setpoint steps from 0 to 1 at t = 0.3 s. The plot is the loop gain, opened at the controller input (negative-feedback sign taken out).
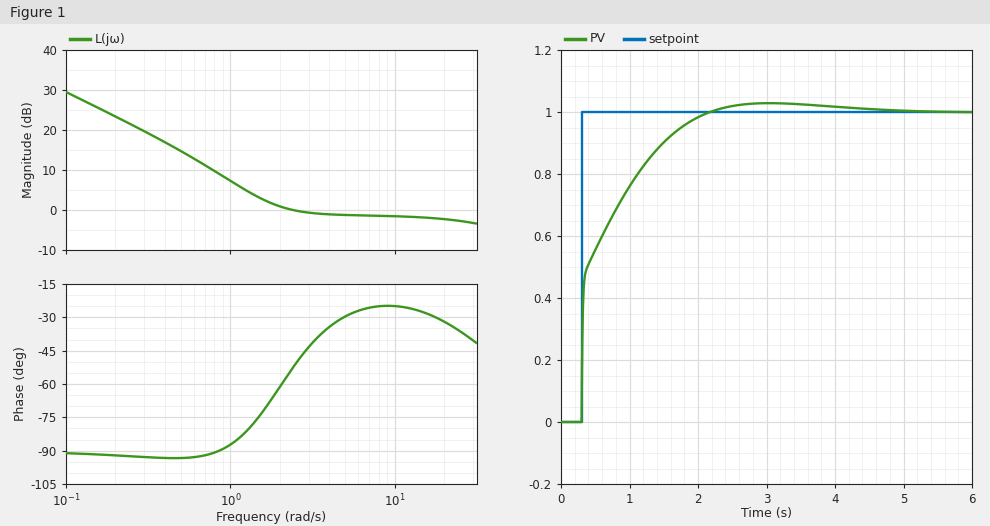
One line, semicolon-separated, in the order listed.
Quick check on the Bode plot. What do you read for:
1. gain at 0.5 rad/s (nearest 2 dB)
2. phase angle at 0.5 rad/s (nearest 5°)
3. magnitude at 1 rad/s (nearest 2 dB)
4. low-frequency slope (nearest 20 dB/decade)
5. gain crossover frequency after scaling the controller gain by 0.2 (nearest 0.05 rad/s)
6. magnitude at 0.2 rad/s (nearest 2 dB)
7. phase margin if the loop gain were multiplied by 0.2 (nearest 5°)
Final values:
14 dB; -95°; 8 dB; -20 dB/decade; 0.55 rad/s; 24 dB; 85°
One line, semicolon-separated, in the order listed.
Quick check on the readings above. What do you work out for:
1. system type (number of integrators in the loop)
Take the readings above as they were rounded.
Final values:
1
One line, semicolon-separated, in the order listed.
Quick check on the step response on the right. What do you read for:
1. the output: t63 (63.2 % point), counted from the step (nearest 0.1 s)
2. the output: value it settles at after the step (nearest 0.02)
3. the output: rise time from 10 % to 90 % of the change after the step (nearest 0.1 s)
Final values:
0.4 s; 1.00; 1.2 s
